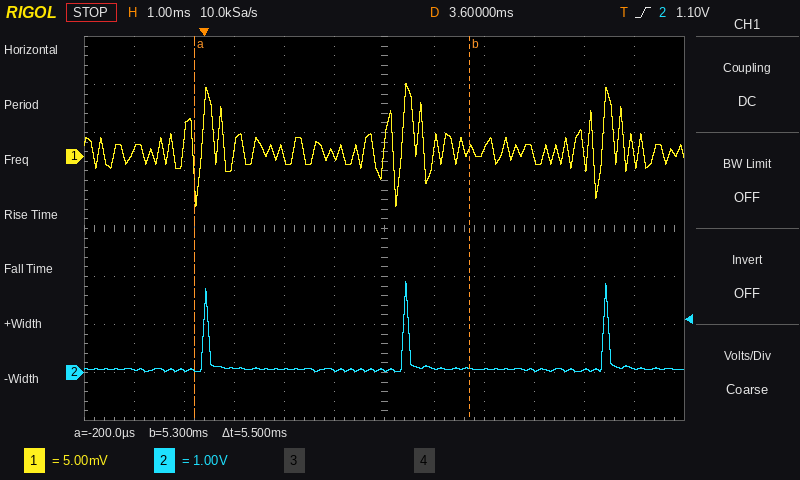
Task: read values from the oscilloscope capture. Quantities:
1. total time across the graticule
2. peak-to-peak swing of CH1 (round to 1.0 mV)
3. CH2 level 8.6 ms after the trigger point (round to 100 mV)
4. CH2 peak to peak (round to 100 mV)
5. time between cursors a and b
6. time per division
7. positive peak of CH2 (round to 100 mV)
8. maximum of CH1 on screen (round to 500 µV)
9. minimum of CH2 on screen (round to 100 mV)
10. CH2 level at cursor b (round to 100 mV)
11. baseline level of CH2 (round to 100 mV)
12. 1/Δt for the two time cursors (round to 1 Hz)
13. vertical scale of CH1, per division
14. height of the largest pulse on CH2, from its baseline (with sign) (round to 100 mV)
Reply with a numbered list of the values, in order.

1. 12 ms
2. 13.0 mV
3. 100 mV
4. 1.9 V
5. 5.5 ms
6. 1 ms
7. 1.9 V
8. 7.5 mV
9. 0.0 V
10. 100 mV
11. 100 mV
12. 182 Hz
13. 5 mV
14. +1.8 V
